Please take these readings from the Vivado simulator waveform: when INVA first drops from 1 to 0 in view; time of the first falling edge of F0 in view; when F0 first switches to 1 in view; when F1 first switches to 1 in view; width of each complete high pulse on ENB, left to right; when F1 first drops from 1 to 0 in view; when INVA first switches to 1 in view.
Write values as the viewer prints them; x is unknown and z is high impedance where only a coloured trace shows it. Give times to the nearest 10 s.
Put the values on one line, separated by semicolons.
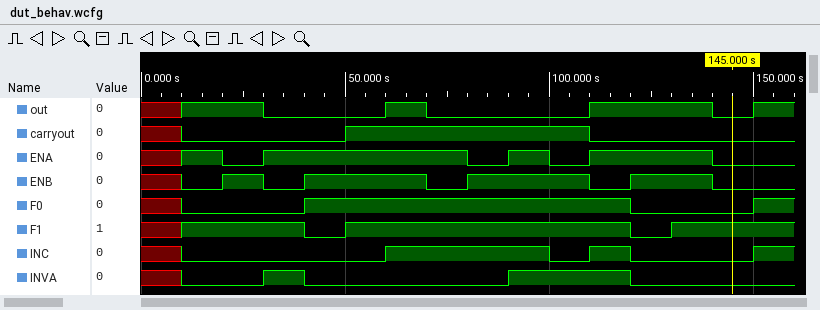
40 s; 120 s; 40 s; 10 s; 10 s, 30 s, 30 s, 20 s; 40 s; 30 s
